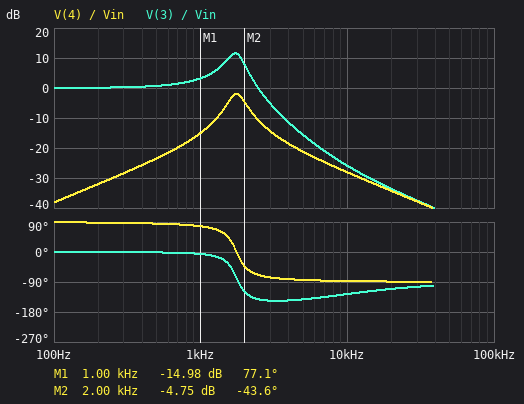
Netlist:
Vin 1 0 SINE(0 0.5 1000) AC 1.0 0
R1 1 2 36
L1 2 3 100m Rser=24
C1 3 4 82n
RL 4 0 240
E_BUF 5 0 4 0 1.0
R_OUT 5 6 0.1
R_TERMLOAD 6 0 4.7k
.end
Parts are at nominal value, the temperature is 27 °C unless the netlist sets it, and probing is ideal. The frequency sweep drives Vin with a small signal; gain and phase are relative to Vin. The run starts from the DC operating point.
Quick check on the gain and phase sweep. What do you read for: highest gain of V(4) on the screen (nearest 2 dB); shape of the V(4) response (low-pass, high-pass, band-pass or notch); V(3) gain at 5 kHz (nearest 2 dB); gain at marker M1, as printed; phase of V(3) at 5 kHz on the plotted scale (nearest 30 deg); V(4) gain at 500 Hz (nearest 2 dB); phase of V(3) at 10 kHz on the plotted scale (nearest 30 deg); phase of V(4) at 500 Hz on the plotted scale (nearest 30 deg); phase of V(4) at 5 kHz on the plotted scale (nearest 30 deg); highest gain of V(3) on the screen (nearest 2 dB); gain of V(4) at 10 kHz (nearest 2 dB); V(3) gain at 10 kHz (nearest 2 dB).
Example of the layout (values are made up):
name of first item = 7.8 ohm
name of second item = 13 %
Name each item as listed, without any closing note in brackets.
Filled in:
highest gain of V(4) on the screen = -2 dB
shape of the V(4) response = band-pass
V(3) gain at 5 kHz = -16 dB
gain at marker M1, as printed = -14.98 dB
phase of V(3) at 5 kHz on the plotted scale = -150 deg
V(4) gain at 500 Hz = -24 dB
phase of V(3) at 10 kHz on the plotted scale = -120 deg
phase of V(4) at 500 Hz on the plotted scale = 90 deg
phase of V(4) at 5 kHz on the plotted scale = -90 deg
highest gain of V(3) on the screen = 12 dB
gain of V(4) at 10 kHz = -28 dB
V(3) gain at 10 kHz = -26 dB
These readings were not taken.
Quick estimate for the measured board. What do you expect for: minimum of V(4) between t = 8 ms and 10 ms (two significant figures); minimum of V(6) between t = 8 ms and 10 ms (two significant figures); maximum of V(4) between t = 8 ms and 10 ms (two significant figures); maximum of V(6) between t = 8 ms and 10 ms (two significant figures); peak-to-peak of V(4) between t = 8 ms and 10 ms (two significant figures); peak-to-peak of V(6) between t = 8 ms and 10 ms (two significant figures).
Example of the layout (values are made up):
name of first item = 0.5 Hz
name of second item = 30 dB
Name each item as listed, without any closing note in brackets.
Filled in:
minimum of V(4) between t = 8 ms and 10 ms = -89 mV
minimum of V(6) between t = 8 ms and 10 ms = -89 mV
maximum of V(4) between t = 8 ms and 10 ms = 89 mV
maximum of V(6) between t = 8 ms and 10 ms = 89 mV
peak-to-peak of V(4) between t = 8 ms and 10 ms = 180 mV
peak-to-peak of V(6) between t = 8 ms and 10 ms = 180 mV
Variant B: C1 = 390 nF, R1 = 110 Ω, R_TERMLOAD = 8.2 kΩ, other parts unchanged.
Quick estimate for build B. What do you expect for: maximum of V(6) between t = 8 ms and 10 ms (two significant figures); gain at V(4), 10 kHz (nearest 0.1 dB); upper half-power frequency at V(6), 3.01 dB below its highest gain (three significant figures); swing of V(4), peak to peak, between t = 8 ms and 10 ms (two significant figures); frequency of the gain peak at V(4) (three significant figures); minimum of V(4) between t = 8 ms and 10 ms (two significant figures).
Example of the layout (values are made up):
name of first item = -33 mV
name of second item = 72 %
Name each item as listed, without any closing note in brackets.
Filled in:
maximum of V(6) between t = 8 ms and 10 ms = 280 mV
gain at V(4), 10 kHz = -28.3 dB
upper half-power frequency at V(6), 3.01 dB below its highest gain = 1.16 kHz
swing of V(4), peak to peak, between t = 8 ms and 10 ms = 550 mV
frequency of the gain peak at V(4) = 806 Hz
minimum of V(4) between t = 8 ms and 10 ms = -280 mV
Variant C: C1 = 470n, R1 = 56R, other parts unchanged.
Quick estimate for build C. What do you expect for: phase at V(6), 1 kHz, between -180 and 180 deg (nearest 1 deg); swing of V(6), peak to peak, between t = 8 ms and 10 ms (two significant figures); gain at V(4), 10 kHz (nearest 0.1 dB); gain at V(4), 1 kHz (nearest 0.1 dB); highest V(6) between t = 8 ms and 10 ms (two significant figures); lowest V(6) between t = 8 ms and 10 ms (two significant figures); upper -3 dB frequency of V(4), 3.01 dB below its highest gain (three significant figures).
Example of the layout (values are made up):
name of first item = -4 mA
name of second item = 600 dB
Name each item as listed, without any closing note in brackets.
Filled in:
phase at V(6), 1 kHz, between -180 and 180 deg = -42 deg
swing of V(6), peak to peak, between t = 8 ms and 10 ms = 560 mV
gain at V(4), 10 kHz = -28.3 dB
gain at V(4), 1 kHz = -5.1 dB
highest V(6) between t = 8 ms and 10 ms = 280 mV
lowest V(6) between t = 8 ms and 10 ms = -280 mV
upper -3 dB frequency of V(4), 3.01 dB below its highest gain = 1.03 kHz
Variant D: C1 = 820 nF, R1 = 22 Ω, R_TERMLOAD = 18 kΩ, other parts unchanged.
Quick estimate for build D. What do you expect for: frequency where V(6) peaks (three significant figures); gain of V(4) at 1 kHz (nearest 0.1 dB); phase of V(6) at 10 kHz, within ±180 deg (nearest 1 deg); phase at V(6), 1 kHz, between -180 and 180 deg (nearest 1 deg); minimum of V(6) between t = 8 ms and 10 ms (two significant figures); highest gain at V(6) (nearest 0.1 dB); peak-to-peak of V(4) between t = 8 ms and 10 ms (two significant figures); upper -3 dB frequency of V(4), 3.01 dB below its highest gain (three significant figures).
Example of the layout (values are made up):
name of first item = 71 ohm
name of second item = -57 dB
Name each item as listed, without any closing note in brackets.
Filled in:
frequency where V(6) peaks = 556 Hz
gain of V(4) at 1 kHz = -6.7 dB
phase of V(6) at 10 kHz, within ±180 deg = -87 deg
phase at V(6), 1 kHz, between -180 and 180 deg = -57 deg
minimum of V(6) between t = 8 ms and 10 ms = -230 mV
highest gain at V(6) = -1.5 dB
peak-to-peak of V(4) between t = 8 ms and 10 ms = 460 mV
upper -3 dB frequency of V(4), 3.01 dB below its highest gain = 828 Hz
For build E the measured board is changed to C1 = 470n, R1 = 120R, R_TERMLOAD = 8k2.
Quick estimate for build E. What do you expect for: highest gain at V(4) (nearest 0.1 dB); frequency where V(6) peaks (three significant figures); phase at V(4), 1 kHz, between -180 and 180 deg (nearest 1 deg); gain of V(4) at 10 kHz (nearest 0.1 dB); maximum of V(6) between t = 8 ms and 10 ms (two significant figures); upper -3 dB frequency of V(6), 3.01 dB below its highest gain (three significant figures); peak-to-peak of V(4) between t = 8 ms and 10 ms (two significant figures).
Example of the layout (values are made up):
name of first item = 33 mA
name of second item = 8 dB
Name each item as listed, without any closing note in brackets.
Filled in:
highest gain at V(4) = -4.1 dB
frequency where V(6) peaks = 734 Hz
phase at V(4), 1 kHz, between -180 and 180 deg = -37 deg
gain of V(4) at 10 kHz = -28.3 dB
maximum of V(6) between t = 8 ms and 10 ms = 250 mV
upper -3 dB frequency of V(6), 3.01 dB below its highest gain = 1.10 kHz
peak-to-peak of V(4) between t = 8 ms and 10 ms = 500 mV
